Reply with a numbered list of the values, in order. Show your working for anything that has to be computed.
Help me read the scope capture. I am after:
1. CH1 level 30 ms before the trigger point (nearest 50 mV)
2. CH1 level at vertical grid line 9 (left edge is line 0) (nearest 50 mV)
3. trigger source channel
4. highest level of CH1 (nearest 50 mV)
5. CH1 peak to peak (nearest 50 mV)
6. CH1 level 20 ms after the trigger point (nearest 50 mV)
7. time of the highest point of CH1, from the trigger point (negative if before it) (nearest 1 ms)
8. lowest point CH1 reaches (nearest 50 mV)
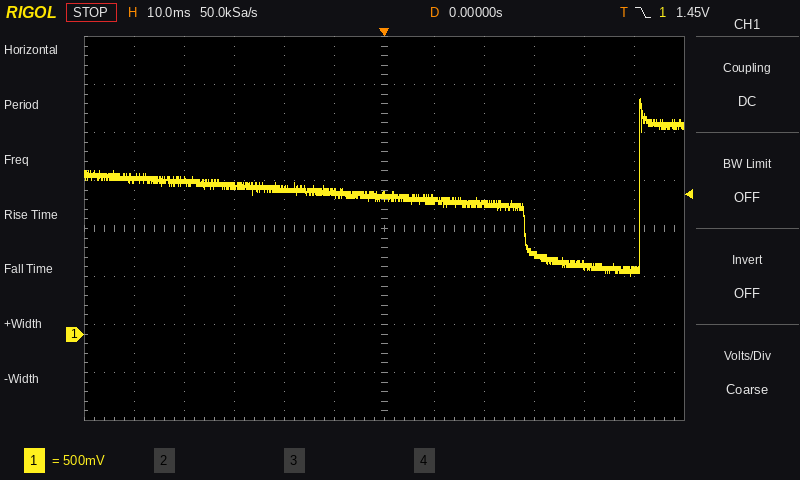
1. 1.55 V
2. 850 mV
3. CH1
4. 2.45 V
5. 2.45 V − (600 mV) = 1.85 V
6. 1.35 V
7. +51 ms
8. 600 mV
